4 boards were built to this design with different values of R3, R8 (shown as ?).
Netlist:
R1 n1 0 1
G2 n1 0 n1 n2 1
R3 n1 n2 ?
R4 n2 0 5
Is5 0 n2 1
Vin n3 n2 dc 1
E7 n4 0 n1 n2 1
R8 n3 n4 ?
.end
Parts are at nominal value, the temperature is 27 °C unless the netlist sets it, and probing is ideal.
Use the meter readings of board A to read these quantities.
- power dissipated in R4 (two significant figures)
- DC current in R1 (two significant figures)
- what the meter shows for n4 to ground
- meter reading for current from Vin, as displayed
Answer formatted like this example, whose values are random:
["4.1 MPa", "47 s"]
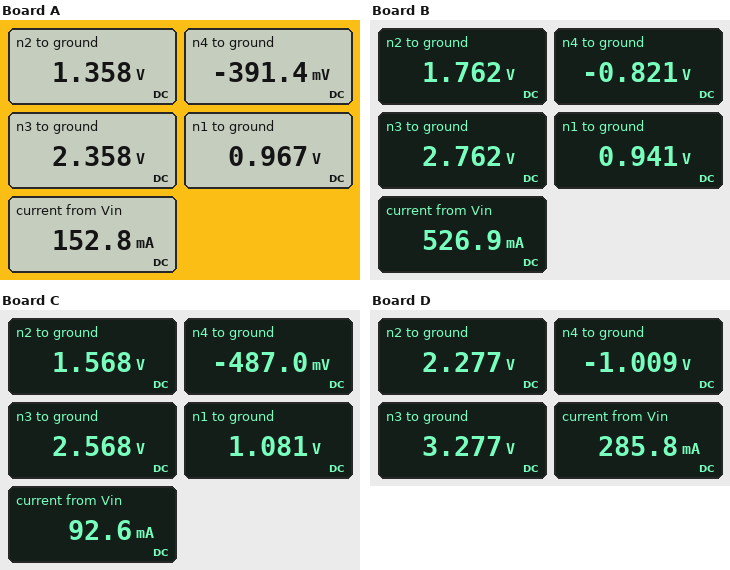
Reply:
["370 mW", "970 mA", "-391.4 mV", "152.8 mA"]
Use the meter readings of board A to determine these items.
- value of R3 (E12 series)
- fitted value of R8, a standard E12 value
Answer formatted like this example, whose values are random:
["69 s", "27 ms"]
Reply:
["0.68 Ω", "18 Ω"]
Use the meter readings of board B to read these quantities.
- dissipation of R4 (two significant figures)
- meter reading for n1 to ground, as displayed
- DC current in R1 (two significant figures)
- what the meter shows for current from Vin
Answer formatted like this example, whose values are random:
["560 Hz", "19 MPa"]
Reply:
["620 mW", "0.941 V", "940 mA", "526.9 mA"]
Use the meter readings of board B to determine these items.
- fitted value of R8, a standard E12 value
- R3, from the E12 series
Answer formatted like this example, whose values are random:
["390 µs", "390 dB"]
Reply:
["6.8 Ω", "6.8 Ω"]
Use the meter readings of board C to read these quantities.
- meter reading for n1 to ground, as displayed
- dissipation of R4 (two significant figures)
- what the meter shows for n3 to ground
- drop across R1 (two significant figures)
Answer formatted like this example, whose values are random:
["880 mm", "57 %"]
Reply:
["1.081 V", "490 mW", "2.568 V", "1.1 V"]
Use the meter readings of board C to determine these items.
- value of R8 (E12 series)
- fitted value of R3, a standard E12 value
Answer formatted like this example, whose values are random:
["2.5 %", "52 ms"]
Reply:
["33 Ω", "0.82 Ω"]
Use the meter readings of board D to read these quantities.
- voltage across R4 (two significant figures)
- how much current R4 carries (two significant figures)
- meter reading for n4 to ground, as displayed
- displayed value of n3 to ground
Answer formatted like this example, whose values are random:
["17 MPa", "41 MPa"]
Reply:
["2.3 V", "460 mA", "-1.009 V", "3.277 V"]
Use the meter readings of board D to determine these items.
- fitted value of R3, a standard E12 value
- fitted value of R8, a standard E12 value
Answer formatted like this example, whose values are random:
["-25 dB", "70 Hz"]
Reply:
["3.9 Ω", "15 Ω"]
